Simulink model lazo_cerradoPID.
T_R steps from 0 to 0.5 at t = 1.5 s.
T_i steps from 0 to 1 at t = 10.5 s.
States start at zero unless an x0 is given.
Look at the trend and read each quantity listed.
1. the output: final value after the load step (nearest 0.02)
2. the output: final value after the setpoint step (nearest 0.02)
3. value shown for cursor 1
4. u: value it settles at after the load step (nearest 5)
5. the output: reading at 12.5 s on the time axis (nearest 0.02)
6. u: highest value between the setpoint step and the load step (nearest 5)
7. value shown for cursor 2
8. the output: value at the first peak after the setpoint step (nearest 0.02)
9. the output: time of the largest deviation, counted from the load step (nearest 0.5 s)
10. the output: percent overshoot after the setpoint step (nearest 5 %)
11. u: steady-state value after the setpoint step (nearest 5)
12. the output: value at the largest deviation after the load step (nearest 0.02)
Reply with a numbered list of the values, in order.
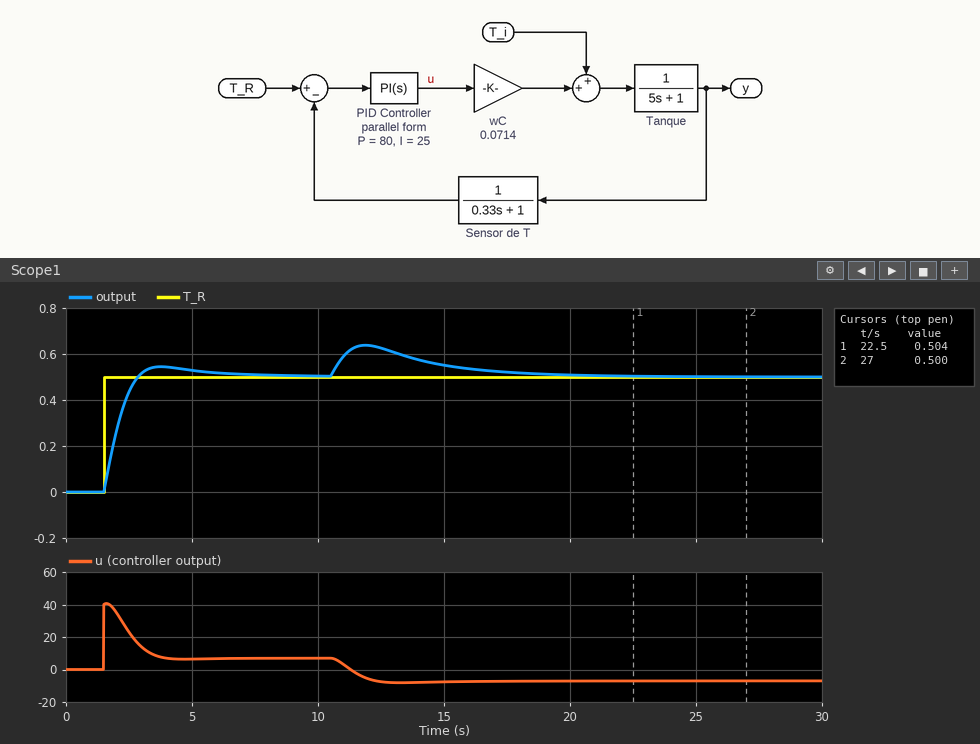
1. 0.50
2. 0.50
3. 0.504
4. -5
5. 0.62
6. 40
7. 0.500
8. 0.54
9. 1.5 s
10. 10 %
11. 5
12. 0.64
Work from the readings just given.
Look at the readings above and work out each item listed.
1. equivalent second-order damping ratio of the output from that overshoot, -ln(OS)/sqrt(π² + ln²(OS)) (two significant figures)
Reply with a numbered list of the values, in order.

1. 0.59
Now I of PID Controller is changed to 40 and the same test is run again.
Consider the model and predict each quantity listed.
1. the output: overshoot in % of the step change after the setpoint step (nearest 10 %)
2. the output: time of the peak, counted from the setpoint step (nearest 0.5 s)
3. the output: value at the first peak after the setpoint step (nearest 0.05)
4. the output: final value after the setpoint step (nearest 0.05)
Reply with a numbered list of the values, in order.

1. 20 %
2. 2.0 s
3. 0.60
4. 0.50
